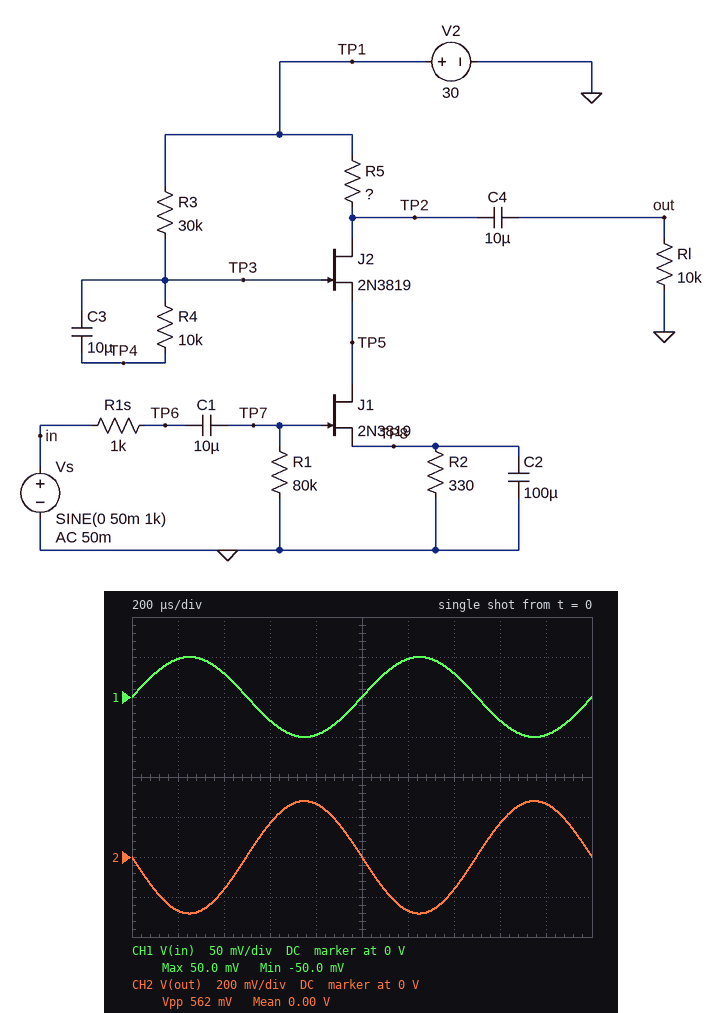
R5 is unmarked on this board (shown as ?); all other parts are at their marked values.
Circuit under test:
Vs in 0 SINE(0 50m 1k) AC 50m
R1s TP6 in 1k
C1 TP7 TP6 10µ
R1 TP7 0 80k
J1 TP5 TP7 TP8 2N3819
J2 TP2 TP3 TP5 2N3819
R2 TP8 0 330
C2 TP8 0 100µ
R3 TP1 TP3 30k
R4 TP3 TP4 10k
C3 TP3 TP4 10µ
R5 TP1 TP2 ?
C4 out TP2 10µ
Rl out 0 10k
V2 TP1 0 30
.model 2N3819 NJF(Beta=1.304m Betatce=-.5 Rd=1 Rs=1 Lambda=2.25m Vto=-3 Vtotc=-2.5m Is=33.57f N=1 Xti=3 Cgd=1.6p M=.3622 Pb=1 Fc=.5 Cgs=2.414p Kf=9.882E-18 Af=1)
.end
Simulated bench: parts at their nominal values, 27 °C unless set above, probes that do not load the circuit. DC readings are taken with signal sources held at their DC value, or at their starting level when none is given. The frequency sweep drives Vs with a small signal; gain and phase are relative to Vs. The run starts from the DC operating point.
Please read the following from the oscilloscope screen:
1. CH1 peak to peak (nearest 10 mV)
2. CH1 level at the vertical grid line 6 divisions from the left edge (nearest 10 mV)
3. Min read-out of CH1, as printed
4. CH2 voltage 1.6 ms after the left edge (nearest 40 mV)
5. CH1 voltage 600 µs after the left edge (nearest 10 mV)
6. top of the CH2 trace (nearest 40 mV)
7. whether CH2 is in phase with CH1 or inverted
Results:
100 mV
50 mV
-50.0 mV
160 mV
-30 mV
280 mV
inverted
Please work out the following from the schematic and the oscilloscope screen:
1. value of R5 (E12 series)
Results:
1.5 kΩ
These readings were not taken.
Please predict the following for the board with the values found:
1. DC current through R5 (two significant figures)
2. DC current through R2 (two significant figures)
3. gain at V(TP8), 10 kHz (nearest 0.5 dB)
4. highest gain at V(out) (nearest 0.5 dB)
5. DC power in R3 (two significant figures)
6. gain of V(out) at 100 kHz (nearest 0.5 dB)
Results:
3.8 mA
3.9 mA
-63.0 dB
15.0 dB
1.0 mW
15.0 dB
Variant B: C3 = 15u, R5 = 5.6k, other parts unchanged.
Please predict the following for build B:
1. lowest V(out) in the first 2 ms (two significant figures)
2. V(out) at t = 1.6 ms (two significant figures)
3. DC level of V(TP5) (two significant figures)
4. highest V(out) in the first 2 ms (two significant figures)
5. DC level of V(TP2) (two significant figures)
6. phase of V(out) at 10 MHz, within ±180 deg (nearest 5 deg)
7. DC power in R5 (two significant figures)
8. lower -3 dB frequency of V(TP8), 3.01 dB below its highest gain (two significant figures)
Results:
-700 mV
420 mV
11 V
690 mV
12 V
145 deg
61 mW
190 mHz
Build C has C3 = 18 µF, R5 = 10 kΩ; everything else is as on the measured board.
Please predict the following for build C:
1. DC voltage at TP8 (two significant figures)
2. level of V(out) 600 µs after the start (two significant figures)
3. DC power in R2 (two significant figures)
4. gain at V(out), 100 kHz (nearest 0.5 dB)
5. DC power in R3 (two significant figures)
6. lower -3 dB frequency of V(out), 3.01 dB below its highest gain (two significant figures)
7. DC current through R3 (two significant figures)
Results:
1.2 V
46 mV
4.4 mW
3.0 dB
24 mW
2.1 Hz
900 µA
